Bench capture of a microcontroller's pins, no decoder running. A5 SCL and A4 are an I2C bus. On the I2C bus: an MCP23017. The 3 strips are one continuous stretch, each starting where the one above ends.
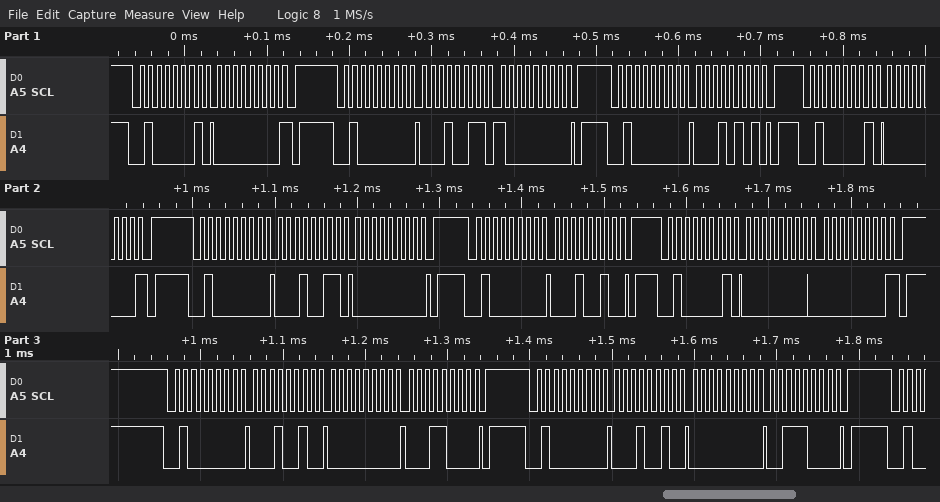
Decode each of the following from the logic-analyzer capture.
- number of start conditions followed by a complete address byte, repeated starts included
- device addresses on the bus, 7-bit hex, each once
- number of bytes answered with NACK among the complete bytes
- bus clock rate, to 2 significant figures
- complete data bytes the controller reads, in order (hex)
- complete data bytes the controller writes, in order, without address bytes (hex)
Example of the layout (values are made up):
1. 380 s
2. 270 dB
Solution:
1. 9
2. 0x20
3. 3
4. 100 kHz
5. 00 00 00 00
6. 13 80 15 13 00 12 12 00 18 12 00 38
